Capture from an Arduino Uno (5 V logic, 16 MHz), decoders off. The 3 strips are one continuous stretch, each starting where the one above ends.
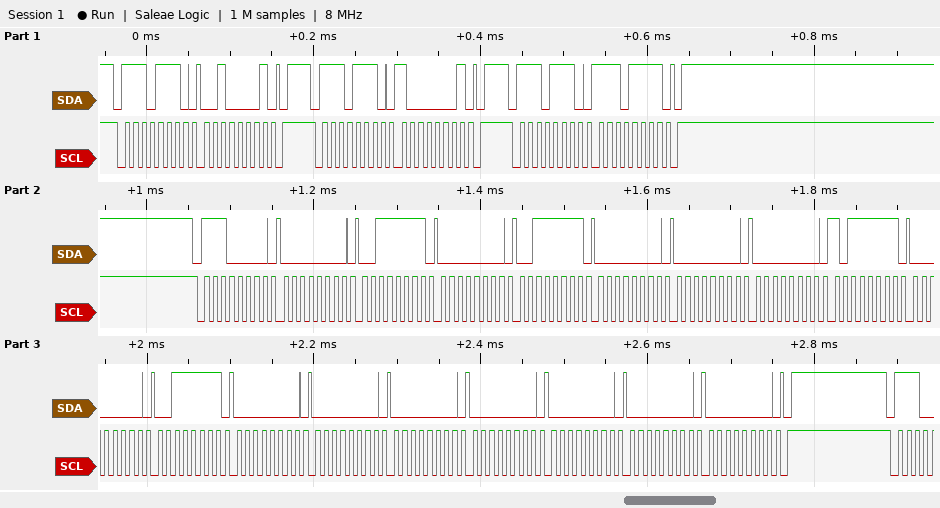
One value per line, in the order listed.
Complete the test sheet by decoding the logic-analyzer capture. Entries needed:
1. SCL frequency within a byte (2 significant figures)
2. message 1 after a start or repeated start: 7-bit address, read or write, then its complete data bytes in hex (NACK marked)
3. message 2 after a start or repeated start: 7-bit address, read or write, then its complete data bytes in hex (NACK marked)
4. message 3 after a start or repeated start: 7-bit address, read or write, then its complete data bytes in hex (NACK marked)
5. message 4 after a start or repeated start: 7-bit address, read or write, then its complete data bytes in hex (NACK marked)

100 kHz
0x77 write: 21
0x77 write: 81
0x77 write: EF
0x70 write: 00 3F 00 3F 00 00 00 BF 00 3F 00 00 00 00 00 00 00
